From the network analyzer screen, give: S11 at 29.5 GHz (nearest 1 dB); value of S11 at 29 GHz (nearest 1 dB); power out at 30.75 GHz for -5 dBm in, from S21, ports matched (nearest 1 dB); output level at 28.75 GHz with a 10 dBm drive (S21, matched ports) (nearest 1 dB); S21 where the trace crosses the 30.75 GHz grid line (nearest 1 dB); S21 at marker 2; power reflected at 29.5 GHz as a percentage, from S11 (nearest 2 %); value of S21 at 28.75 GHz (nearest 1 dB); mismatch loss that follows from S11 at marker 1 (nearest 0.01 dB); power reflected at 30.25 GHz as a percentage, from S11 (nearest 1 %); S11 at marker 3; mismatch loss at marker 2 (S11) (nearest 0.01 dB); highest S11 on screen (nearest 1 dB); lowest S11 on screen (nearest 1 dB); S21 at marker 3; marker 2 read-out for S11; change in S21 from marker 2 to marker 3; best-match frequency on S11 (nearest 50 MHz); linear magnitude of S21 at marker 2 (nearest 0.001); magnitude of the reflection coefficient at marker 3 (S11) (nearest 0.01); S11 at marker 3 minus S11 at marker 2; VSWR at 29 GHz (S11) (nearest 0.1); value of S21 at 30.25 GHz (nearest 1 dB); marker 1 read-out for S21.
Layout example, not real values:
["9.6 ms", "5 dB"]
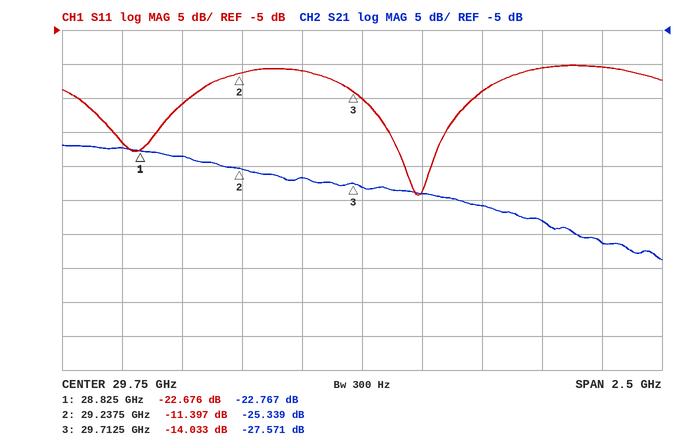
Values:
["-11 dB", "-16 dB", "-41 dBm", "-12 dBm", "-36 dB", "-25.339 dB", "8 %", "-22 dB", "0.02 dB", "4 %", "-14.033 dB", "0.33 dB", "-10 dB", "-29 dB", "-27.571 dB", "-11.397 dB", "-2.232 dB", "30.00 GHz", "0.054", "0.20", "-2.636 dB", "1.4", "-31 dB", "-22.767 dB"]
